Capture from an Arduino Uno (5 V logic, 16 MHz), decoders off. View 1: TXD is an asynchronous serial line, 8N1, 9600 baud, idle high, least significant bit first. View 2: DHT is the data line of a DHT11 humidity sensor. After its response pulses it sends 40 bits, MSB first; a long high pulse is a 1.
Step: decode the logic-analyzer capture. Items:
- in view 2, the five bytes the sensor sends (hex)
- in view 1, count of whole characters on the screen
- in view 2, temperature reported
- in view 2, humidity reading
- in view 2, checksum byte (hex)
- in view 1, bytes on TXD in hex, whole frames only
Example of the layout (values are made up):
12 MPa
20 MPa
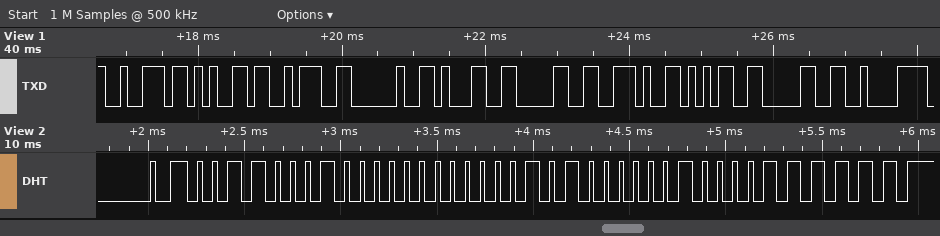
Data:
31 00 0A 04 3F
10
10.4 °C
49 %
0x3F
72 65 3A 20 31 30 2E 35 30 C2
